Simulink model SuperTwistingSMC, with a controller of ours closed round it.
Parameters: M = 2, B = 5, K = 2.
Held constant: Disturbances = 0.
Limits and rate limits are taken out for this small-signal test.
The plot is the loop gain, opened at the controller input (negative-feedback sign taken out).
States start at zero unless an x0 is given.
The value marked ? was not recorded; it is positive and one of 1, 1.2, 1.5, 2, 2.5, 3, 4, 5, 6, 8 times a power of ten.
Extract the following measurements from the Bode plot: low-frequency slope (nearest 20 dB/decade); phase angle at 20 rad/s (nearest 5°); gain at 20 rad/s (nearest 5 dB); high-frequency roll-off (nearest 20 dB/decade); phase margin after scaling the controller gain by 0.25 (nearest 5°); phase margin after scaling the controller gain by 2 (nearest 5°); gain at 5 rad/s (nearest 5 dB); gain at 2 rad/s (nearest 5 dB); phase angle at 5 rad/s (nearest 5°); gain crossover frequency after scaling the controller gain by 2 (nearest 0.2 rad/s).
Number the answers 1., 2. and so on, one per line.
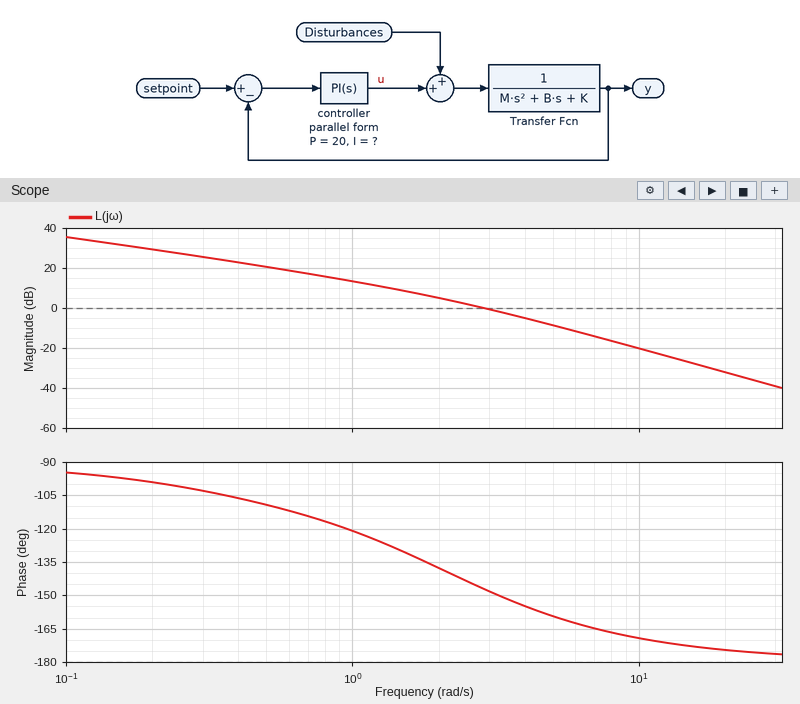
1. -20 dB/decade
2. -175°
3. -30 dB
4. -40 dB/decade
5. 55°
6. 25°
7. -10 dB
8. 5 dB
9. -160°
10. 4.2 rad/s
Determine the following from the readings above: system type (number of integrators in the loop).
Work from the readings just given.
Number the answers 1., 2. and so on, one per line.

1. 1
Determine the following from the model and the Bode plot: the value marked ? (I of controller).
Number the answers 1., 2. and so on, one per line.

1. 12
